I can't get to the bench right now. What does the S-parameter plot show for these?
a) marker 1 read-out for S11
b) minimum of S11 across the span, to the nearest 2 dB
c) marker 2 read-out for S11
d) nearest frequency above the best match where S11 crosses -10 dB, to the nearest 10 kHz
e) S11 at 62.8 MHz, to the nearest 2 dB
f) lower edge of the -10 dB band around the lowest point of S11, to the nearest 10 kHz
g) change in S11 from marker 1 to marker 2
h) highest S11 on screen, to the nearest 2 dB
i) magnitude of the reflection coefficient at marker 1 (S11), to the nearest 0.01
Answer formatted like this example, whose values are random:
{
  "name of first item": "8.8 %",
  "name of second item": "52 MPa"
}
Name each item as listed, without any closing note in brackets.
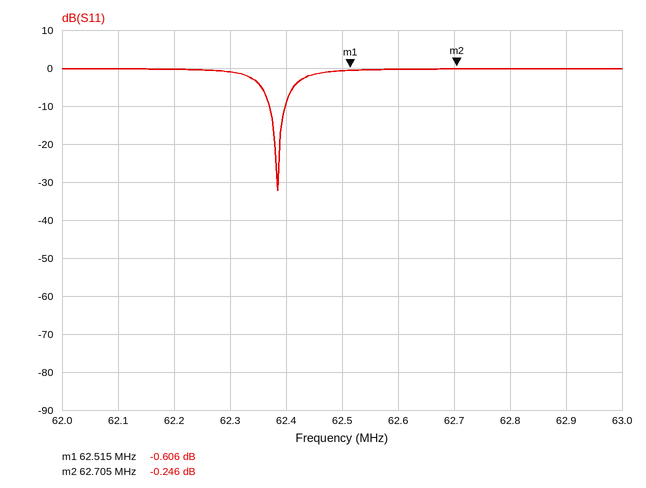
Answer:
{
  "marker 1 read-out for S11": "-0.606 dB",
  "minimum of S11 across the span, to the nearest 2 dB": "-32 dB",
  "marker 2 read-out for S11": "-0.246 dB",
  "nearest frequency above the best match where S11 crosses -10 dB, to the nearest 10 kHz": "62.40 MHz",
  "S11 at 62.8 MHz, to the nearest 2 dB": "0 dB",
  "lower edge of the -10 dB band around the lowest point of S11, to the nearest 10 kHz": "62.37 MHz",
  "change in S11 from marker 1 to marker 2": "0.360 dB",
  "highest S11 on screen, to the nearest 2 dB": "0 dB",
  "magnitude of the reflection coefficient at marker 1 (S11), to the nearest 0.01": "0.93"
}
